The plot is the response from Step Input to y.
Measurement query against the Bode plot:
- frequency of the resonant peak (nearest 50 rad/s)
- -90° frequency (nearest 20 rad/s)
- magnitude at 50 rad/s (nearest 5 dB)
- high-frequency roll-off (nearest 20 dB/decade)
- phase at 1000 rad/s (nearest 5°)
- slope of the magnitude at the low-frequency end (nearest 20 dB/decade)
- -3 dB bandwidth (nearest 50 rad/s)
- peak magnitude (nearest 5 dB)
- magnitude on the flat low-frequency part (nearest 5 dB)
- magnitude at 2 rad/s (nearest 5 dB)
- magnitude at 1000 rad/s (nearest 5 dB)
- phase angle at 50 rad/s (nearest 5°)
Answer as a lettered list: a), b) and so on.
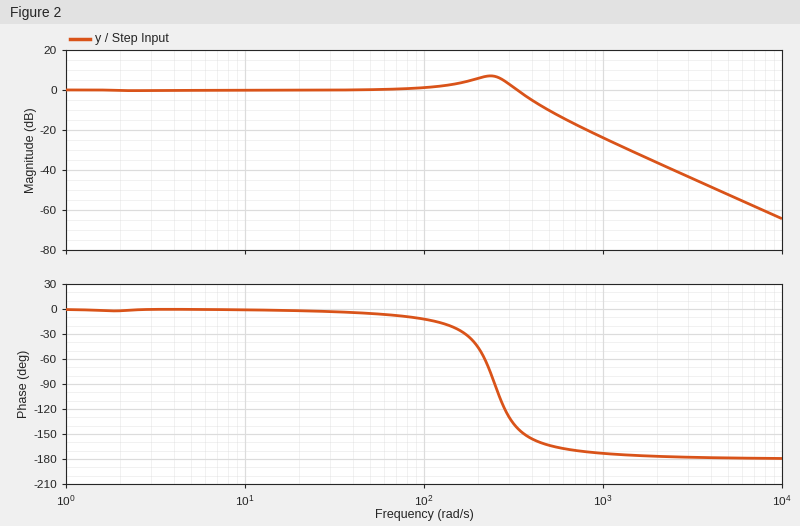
a) 250 rad/s
b) 240 rad/s
c) 0 dB
d) -40 dB/decade
e) -175°
f) 0 dB/decade
g) 350 rad/s
h) 5 dB
i) 0 dB
j) 0 dB
k) -25 dB
l) -5°
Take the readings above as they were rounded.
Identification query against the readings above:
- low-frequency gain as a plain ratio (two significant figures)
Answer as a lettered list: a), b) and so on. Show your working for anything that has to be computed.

a) 10^(0 / 20) = 1.0
